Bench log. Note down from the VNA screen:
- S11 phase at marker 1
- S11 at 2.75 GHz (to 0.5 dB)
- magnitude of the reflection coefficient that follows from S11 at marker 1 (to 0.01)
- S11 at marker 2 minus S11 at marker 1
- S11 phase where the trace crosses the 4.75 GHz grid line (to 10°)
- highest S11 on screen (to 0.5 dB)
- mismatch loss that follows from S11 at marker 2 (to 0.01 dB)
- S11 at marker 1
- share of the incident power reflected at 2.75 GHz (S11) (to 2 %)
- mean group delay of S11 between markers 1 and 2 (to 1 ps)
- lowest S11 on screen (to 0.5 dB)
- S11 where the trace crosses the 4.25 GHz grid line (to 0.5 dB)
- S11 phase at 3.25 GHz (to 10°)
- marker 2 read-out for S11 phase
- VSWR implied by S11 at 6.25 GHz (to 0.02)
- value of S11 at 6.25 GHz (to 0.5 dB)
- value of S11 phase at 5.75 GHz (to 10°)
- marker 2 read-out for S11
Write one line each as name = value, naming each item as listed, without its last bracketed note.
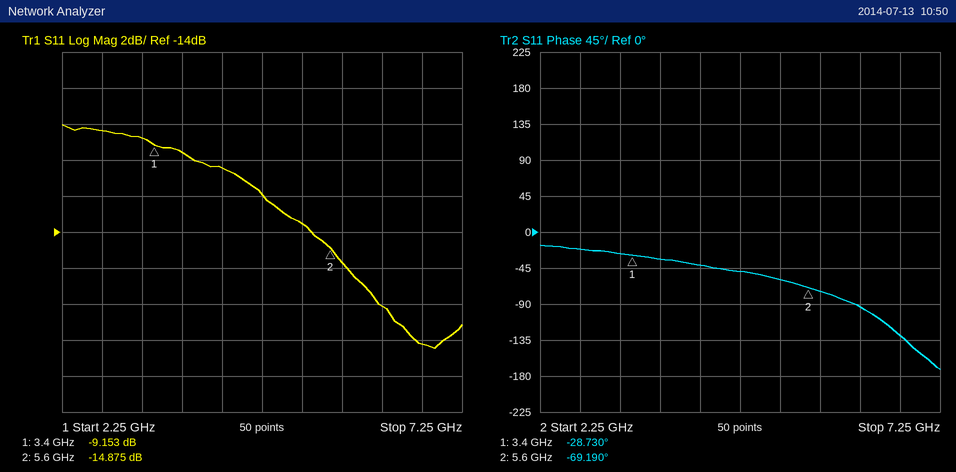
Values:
S11 phase at marker 1 = -28.730°
S11 at 2.75 GHz = -8.5 dB
magnitude of the reflection coefficient that follows from S11 at marker 1 = 0.35
S11 at marker 2 minus S11 at marker 1 = -5.722 dB
S11 phase where the trace crosses the 4.75 GHz grid line = -50°
highest S11 on screen = -8.0 dB
mismatch loss that follows from S11 at marker 2 = 0.14 dB
S11 at marker 1 = -9.153 dB
share of the incident power reflected at 2.75 GHz (S11) = 14 %
mean group delay of S11 between markers 1 and 2 = 51 ps
lowest S11 on screen = -20.5 dB
S11 where the trace crosses the 4.25 GHz grid line = -10.5 dB
S11 phase at 3.25 GHz = -30°
marker 2 read-out for S11 phase = -69.190°
VSWR implied by S11 at 6.25 GHz = 1.28
value of S11 at 6.25 GHz = -18.0 dB
value of S11 phase at 5.75 GHz = -70°
marker 2 read-out for S11 = -14.875 dB
